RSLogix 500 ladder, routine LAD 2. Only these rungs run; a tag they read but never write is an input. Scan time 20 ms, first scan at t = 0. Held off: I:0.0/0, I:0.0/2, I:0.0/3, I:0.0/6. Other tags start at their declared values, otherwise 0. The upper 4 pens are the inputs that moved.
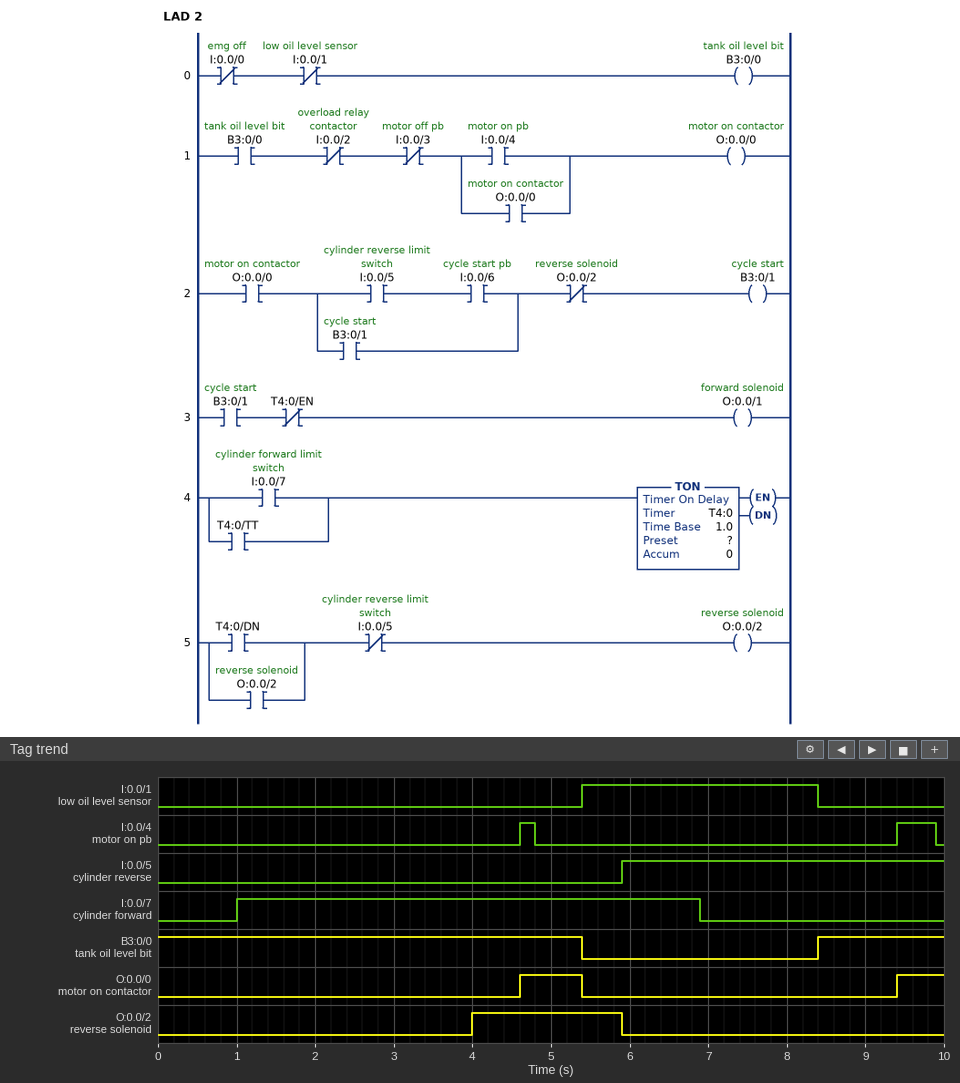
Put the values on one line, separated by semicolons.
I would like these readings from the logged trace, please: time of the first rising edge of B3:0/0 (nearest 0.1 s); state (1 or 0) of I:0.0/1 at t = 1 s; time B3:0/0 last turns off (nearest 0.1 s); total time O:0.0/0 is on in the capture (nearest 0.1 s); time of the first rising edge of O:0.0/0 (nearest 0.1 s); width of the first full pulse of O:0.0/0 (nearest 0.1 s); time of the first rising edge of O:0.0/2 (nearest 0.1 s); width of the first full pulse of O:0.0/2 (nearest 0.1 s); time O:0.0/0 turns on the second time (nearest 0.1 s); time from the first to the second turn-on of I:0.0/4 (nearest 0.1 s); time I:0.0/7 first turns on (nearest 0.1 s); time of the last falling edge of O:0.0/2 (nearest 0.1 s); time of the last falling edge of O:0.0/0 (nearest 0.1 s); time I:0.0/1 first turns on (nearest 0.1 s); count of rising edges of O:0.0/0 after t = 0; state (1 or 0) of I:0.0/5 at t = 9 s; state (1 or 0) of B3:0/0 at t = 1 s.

8.4 s; 0; 5.4 s; 1.4 s; 4.6 s; 0.8 s; 4.0 s; 1.9 s; 9.4 s; 4.8 s; 1.0 s; 5.9 s; 5.4 s; 5.4 s; 2; 1; 1
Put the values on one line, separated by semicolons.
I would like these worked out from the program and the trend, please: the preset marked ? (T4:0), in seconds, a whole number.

3 s
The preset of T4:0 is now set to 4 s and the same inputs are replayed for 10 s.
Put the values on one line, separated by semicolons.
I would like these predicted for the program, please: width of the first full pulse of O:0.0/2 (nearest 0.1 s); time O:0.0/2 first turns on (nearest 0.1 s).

0.9 s; 5.0 s
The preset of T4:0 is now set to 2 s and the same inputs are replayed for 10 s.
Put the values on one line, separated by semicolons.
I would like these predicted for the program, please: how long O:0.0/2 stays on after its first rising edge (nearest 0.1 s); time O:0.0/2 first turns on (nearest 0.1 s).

2.9 s; 3.0 s
